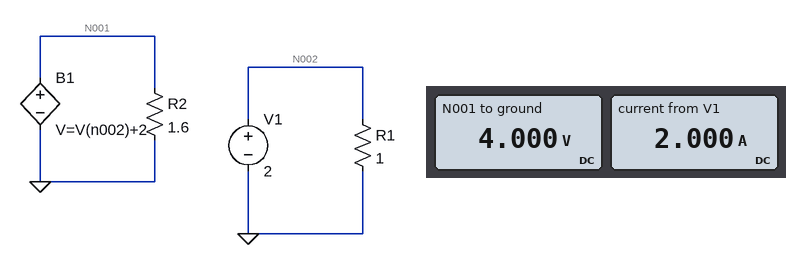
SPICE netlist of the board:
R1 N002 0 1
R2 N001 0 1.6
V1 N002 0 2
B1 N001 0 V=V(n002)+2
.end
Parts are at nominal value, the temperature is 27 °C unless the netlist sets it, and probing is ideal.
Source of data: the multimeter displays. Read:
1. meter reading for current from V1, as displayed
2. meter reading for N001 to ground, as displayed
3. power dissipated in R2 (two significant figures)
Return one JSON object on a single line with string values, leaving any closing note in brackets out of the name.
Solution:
{"meter reading for current from V1, as displayed": "2.000 A", "meter reading for N001 to ground, as displayed": "4.000 V", "power dissipated in R2": "10 W"}
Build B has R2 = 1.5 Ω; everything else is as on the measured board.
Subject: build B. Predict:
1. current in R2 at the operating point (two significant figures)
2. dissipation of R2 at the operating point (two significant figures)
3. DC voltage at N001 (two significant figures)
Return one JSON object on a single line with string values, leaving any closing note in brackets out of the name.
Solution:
{"current in R2 at the operating point": "2.7 A", "dissipation of R2 at the operating point": "11 W", "DC voltage at N001": "4.0 V"}
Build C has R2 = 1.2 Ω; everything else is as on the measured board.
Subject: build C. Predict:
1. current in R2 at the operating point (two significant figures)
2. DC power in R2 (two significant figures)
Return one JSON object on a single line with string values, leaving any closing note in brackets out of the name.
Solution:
{"current in R2 at the operating point": "3.3 A", "DC power in R2": "13 W"}
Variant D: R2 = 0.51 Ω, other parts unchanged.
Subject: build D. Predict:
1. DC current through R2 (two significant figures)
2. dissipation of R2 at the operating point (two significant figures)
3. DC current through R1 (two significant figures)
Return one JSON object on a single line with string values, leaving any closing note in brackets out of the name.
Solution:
{"DC current through R2": "7.8 A", "dissipation of R2 at the operating point": "31 W", "DC current through R1": "2.0 A"}
